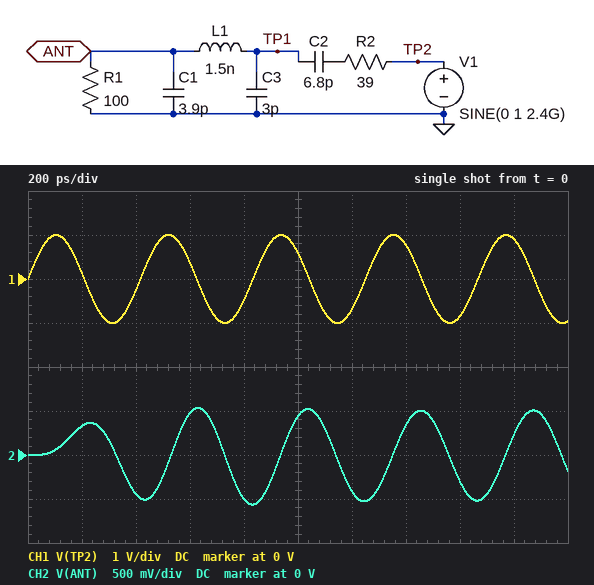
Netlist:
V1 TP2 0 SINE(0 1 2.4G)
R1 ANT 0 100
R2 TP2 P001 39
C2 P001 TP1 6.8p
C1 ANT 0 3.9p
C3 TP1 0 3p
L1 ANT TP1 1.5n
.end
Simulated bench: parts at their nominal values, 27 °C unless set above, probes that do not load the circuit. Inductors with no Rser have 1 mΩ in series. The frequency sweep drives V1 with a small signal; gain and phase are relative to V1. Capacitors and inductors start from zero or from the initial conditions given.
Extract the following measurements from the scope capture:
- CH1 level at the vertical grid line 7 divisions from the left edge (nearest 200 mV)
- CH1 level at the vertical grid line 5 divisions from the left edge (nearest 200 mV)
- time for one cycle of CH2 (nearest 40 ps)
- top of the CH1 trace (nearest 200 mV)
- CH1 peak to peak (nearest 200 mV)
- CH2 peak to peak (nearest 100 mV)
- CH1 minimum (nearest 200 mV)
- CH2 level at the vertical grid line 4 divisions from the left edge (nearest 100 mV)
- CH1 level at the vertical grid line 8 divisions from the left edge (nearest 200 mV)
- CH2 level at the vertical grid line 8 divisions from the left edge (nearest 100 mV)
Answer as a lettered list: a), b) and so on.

a) 800 mV
b) 600 mV
c) 400 ps
d) 1.0 V
e) 2.0 V
f) 1.1 V
g) -1.0 V
h) -500 mV
i) -800 mV
j) -300 mV
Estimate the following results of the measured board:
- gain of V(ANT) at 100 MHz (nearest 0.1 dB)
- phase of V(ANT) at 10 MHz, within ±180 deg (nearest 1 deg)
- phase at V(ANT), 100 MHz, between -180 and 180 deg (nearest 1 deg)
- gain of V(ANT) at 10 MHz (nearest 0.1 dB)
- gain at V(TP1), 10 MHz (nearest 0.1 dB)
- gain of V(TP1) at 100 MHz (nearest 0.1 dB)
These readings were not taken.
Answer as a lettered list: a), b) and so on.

a) -10.2 dB
b) 84 deg
c) 42 deg
d) -27.4 dB
e) -27.4 dB
f) -10.2 dB
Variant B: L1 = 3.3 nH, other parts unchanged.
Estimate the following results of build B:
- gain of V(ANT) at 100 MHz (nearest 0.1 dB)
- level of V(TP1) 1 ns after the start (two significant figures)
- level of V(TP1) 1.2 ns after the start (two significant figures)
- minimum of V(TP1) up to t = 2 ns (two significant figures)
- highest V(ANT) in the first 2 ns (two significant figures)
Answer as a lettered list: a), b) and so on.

a) -10.1 dB
b) 640 mV
c) -710 mV
d) -770 mV
e) 420 mV
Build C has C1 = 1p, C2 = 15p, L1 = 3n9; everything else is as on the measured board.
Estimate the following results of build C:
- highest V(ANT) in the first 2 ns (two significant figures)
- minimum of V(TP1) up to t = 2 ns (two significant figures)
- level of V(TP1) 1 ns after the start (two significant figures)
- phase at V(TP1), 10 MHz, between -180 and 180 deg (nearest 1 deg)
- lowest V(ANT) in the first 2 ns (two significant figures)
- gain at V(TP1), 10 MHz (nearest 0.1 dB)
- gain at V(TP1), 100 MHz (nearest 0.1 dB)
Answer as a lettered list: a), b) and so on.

a) 650 mV
b) -420 mV
c) 340 mV
d) 81 deg
e) -670 mV
f) -20.6 dB
g) -5.6 dB
